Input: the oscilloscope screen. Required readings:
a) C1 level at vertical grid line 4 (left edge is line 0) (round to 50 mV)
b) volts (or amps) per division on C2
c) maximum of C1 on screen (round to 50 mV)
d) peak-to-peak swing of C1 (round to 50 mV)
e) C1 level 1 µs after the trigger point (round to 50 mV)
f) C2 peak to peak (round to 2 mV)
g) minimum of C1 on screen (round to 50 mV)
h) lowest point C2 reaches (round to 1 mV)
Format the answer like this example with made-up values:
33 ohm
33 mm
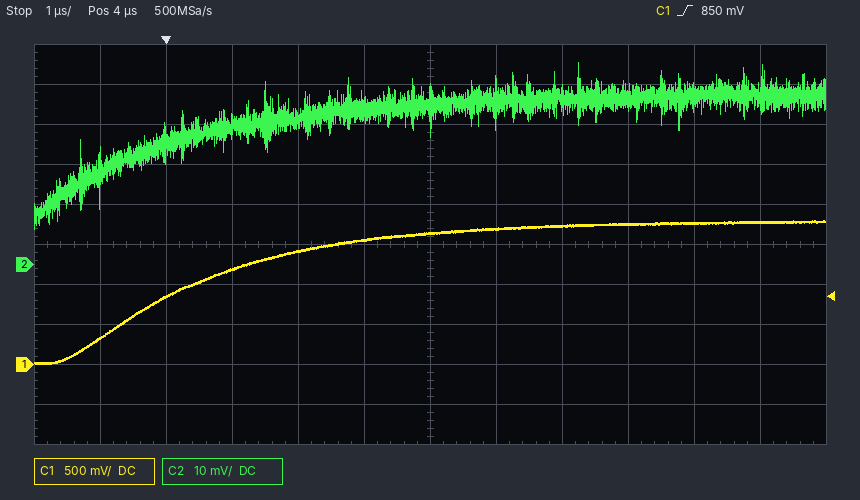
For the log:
1.40 V
10 mV
1.80 V
1.80 V
1.20 V
42 mV
0 mV
9 mV
